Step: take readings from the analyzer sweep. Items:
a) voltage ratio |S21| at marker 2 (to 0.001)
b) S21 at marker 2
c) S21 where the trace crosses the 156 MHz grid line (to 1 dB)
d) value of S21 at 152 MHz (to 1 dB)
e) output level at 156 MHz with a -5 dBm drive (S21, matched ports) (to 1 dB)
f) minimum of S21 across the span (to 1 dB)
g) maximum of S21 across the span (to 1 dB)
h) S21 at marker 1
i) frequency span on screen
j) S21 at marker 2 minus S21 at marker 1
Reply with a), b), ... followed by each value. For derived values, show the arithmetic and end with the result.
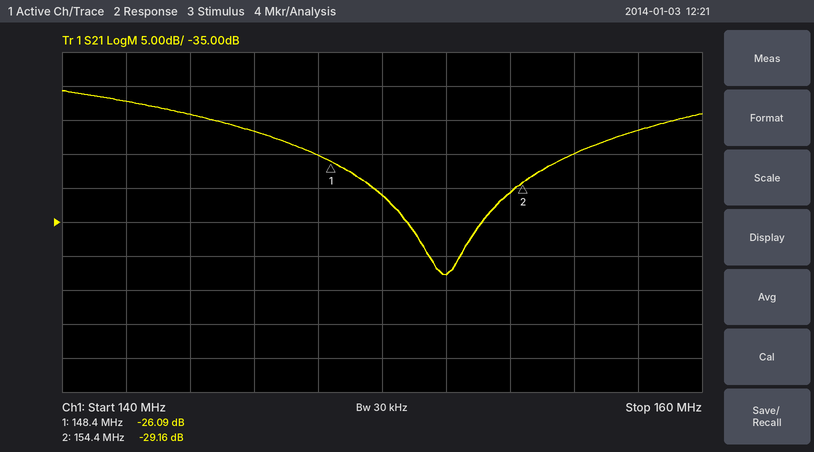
a) 10^(-29.16/20) ≈ 0.035
b) -29.16 dB
c) -25 dB
d) -43 dB
e) -5 dBm + (-25 dB) = -30 dBm
f) -43 dB
g) -16 dB
h) -26.09 dB
i) 20 MHz
j) -29.16 − (-26.09) = -3.07 dB
